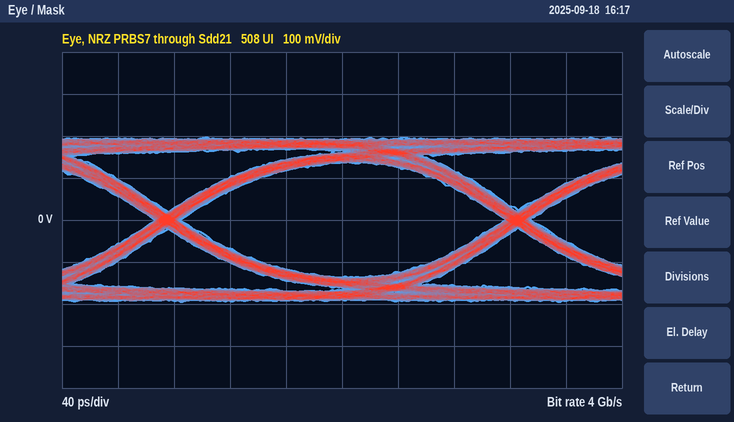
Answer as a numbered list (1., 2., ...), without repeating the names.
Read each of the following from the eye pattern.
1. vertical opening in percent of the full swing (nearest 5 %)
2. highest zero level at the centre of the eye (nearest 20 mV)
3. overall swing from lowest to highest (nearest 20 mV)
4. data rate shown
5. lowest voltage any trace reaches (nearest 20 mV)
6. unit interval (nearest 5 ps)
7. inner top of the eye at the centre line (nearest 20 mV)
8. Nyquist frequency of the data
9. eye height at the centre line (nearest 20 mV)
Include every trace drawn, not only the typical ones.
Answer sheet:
1. 70 %
2. -140 mV
3. 400 mV
4. 4 Gb/s
5. -200 mV
6. 250 ps
7. 140 mV
8. 2 GHz
9. 280 mV
